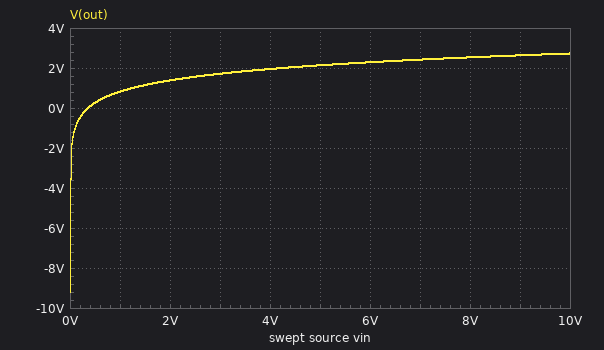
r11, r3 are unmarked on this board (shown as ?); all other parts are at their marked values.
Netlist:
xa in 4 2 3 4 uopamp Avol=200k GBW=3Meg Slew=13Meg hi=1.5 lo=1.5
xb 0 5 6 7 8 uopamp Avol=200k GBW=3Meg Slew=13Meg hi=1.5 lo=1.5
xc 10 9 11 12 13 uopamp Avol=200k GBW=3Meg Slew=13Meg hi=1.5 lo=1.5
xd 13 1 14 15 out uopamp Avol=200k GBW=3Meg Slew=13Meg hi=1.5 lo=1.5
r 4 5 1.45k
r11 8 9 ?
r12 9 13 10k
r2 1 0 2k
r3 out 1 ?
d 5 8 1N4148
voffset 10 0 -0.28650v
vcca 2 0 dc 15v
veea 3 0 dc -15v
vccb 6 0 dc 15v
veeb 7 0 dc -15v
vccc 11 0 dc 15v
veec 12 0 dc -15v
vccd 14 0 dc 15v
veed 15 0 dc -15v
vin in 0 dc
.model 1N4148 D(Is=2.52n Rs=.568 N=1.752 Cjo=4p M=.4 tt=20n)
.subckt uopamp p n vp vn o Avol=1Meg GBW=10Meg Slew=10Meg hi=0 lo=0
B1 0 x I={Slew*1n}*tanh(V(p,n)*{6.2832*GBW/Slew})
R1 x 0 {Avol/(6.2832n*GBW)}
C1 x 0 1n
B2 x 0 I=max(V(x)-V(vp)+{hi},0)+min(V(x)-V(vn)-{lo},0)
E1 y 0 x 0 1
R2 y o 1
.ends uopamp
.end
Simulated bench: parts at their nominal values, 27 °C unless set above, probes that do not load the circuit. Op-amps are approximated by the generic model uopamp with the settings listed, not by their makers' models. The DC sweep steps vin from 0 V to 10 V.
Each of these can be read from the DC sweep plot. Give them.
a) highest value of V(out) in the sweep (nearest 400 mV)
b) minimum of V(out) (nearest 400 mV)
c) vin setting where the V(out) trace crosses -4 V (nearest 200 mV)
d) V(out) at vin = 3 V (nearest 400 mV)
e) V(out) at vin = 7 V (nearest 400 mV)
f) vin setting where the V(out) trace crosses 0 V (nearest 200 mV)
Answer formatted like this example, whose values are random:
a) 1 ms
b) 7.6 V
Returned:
a) 2.8 V
b) -9.2 V
c) 0 V
d) 1.6 V
e) 2.4 V
f) 400 mV
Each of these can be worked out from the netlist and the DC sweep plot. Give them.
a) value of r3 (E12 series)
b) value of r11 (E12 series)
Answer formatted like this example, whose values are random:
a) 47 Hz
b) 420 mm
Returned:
a) 27 kΩ
b) 8.2 kΩ
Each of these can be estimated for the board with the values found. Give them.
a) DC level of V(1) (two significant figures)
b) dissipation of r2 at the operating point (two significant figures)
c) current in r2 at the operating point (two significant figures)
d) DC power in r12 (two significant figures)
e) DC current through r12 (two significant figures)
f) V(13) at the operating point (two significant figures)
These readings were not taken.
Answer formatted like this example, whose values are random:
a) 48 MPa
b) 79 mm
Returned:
a) -640 mV
b) 200 µW
c) 320 µA
d) 12 µW
e) 35 µA
f) -640 mV
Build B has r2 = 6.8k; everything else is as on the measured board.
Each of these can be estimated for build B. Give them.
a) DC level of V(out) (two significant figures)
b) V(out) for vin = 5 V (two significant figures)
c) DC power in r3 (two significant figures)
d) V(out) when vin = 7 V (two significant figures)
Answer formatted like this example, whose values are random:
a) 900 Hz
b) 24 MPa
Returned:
a) -3.2 V
b) 730 mV
c) 240 µW
d) 830 mV
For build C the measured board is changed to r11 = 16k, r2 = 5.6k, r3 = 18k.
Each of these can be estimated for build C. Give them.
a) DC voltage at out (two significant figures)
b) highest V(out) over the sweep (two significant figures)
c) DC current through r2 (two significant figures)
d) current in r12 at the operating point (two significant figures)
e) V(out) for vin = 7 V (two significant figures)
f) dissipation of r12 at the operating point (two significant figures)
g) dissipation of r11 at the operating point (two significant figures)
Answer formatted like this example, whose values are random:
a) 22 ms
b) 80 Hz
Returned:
a) -2.0 V
b) -180 mV
c) 83 µA
d) 18 µA
e) -230 mV
f) 3.2 µW
g) 5.1 µW
